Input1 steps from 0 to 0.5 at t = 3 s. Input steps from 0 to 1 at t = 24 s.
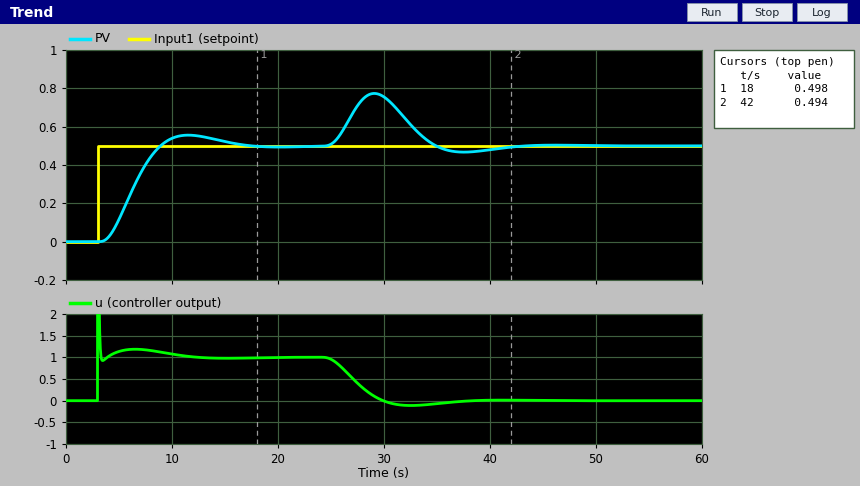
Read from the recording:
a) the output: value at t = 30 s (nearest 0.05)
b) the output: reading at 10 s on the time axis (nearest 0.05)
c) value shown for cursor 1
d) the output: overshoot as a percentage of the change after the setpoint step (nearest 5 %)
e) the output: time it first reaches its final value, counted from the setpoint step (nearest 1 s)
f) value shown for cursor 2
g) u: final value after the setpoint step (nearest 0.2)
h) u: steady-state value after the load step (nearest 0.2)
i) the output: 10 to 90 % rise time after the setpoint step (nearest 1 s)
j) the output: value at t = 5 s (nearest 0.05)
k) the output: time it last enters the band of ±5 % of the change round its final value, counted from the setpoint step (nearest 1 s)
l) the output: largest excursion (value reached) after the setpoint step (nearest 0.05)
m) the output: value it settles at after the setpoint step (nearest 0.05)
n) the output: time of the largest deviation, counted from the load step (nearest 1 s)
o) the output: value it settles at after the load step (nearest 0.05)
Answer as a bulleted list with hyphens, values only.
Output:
- 0.75
- 0.55
- 0.498
- 10 %
- 6 s
- 0.494
- 1.0
- 0.0
- 4 s
- 0.10
- 12 s
- 0.55
- 0.50
- 5 s
- 0.50
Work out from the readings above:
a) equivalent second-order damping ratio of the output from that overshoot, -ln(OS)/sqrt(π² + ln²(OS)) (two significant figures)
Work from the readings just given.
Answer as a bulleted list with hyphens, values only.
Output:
- 0.59
